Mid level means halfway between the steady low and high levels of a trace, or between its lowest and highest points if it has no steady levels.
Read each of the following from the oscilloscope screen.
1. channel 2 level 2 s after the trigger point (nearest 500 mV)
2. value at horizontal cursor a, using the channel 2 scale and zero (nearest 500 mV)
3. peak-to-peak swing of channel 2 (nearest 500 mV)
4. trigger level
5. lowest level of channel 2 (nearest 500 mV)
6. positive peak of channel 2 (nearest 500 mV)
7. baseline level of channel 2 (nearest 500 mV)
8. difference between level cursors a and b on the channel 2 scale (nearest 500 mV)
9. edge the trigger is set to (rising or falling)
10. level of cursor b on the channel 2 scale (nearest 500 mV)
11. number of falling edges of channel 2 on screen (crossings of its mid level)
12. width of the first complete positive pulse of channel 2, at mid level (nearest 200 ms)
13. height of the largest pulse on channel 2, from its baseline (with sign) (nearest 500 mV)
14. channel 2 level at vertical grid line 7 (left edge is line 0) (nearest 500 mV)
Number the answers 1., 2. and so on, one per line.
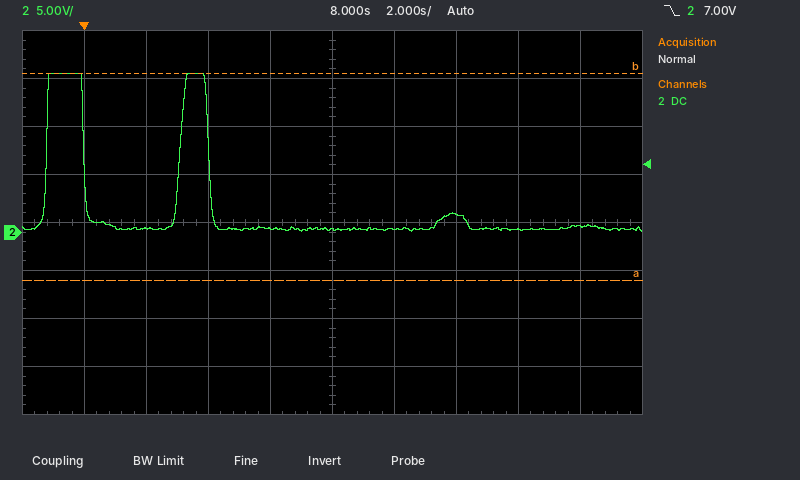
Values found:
1. 500 mV
2. -5.0 V
3. 16.5 V
4. 7.00 V
5. 0.0 V
6. 16.5 V
7. 500 mV
8. 21.5 V
9. falling
10. 16.5 V
11. 2
12. 1.2 s
13. +16.0 V
14. 2.0 V
